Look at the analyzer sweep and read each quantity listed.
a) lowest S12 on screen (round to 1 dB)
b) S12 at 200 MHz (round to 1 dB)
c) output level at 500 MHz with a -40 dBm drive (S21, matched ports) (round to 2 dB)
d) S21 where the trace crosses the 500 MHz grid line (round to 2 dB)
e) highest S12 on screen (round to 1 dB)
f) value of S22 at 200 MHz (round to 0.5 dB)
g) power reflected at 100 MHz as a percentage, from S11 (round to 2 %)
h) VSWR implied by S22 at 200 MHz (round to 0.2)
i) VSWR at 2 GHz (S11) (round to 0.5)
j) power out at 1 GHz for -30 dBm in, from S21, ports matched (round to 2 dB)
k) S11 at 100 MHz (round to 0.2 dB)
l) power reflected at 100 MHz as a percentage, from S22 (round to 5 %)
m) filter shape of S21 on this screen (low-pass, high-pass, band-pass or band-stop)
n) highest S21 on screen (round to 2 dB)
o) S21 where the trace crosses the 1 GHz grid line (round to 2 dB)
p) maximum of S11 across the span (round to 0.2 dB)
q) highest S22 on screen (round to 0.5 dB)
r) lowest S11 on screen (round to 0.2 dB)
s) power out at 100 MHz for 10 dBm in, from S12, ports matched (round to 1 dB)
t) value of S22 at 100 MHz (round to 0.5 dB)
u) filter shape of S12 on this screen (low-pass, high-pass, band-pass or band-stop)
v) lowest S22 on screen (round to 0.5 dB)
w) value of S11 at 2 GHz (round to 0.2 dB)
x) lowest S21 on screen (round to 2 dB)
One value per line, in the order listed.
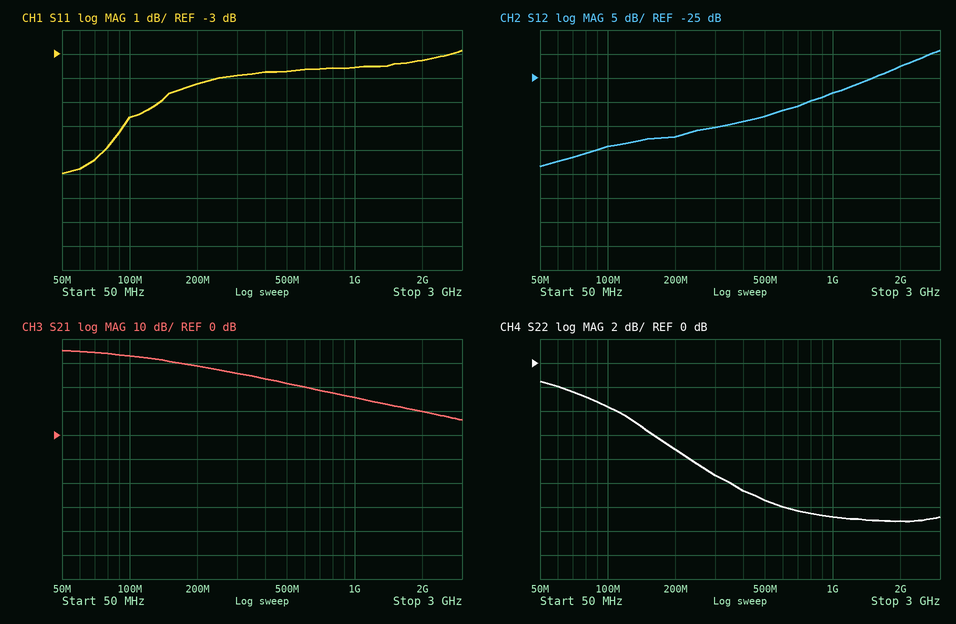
-43 dB
-37 dB
-18 dBm
22 dB
-19 dB
-7.0 dB
28 %
2.6
5.5
-14 dBm
-5.6 dB
45 %
low-pass
36 dB
16 dB
-2.8 dB
-1.5 dB
-8.0 dB
-29 dBm
-3.5 dB
high-pass
-13.0 dB
-3.2 dB
6 dB
